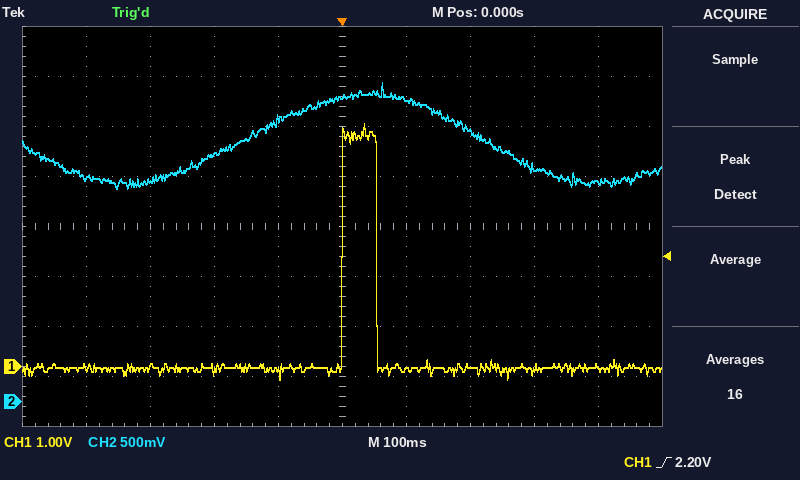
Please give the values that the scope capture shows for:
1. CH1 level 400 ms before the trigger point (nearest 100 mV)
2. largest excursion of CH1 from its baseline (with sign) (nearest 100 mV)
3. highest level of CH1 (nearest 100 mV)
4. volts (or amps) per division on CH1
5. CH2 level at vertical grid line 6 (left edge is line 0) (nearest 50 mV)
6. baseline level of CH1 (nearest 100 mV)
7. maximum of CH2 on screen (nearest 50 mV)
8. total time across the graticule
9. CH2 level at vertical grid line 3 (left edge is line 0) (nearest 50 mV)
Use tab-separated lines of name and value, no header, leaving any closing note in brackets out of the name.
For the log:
CH1 level 400 ms before the trigger point	0.0 V
largest excursion of CH1 from its baseline (with sign)	+4.9 V
highest level of CH1	4.9 V
volts (or amps) per division on CH1	1 V
CH2 level at vertical grid line 6 (left edge is line 0)	3.00 V
baseline level of CH1	0.0 V
maximum of CH2 on screen	3.20 V
total time across the graticule	1 s
CH2 level at vertical grid line 3 (left edge is line 0)	2.45 V
